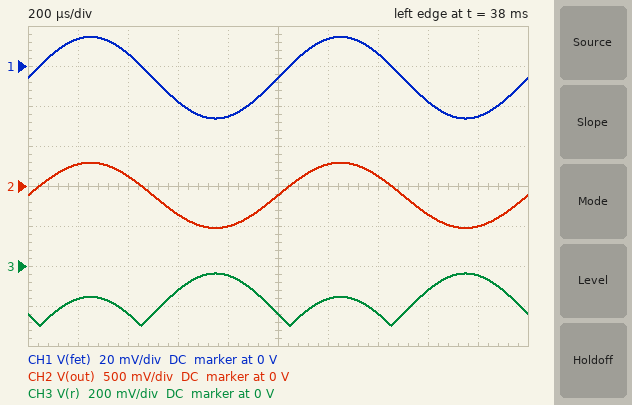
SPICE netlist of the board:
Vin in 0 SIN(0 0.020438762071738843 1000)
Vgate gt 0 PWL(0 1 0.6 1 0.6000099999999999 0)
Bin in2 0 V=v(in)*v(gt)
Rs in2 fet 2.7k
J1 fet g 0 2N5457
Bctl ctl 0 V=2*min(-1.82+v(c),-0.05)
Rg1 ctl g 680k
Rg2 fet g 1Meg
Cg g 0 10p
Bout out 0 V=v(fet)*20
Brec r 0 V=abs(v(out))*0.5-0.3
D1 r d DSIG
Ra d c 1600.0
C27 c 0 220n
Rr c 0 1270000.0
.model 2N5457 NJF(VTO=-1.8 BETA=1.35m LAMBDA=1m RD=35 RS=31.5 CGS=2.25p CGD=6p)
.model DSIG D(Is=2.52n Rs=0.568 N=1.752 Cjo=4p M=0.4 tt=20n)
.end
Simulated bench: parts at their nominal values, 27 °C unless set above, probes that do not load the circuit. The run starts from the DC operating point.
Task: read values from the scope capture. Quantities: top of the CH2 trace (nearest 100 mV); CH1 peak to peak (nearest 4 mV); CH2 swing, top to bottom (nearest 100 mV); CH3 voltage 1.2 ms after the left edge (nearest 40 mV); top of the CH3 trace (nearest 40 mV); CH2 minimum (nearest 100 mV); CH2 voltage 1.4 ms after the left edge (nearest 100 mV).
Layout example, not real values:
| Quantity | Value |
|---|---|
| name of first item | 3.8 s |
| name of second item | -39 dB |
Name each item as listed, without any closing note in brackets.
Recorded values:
| Quantity | Value |
|---|---|
| top of the CH2 trace | 300 mV |
| CH1 peak to peak | 40 mV |
| CH2 swing, top to bottom | 800 mV |
| CH3 voltage 1.2 ms after the left edge | -160 mV |
| top of the CH3 trace | -40 mV |
| CH2 minimum | -500 mV |
| CH2 voltage 1.4 ms after the left edge | 100 mV |
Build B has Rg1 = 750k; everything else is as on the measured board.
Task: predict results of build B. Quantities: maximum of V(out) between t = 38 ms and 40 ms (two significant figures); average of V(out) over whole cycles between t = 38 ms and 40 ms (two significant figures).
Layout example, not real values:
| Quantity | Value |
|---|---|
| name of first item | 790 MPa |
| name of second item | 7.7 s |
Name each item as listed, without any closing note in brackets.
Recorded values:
| Quantity | Value |
|---|---|
| maximum of V(out) between t = 38 ms and 40 ms | 300 mV |
| average of V(out) over whole cycles between t = 38 ms and 40 ms | -110 mV |
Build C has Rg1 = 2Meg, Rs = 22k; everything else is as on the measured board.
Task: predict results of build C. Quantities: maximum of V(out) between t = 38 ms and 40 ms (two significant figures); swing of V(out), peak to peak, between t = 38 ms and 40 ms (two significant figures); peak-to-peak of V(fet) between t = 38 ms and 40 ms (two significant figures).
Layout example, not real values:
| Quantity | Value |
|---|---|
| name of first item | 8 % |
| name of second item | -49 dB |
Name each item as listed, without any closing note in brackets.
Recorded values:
| Quantity | Value |
|---|---|
| maximum of V(out) between t = 38 ms and 40 ms | -3.9 mV |
| swing of V(out), peak to peak, between t = 38 ms and 40 ms | 25 mV |
| peak-to-peak of V(fet) between t = 38 ms and 40 ms | 1.3 mV |
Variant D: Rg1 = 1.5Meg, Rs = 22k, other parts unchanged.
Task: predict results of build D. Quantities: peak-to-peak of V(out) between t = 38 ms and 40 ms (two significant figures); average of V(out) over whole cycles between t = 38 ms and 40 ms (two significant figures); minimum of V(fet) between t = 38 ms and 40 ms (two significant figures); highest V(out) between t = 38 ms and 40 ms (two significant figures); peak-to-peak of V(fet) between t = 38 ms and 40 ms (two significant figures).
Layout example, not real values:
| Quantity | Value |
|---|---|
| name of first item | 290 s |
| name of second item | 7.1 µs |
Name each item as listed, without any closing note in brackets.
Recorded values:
| Quantity | Value |
|---|---|
| peak-to-peak of V(out) between t = 38 ms and 40 ms | 41 mV |
| average of V(out) over whole cycles between t = 38 ms and 40 ms | -32 mV |
| minimum of V(fet) between t = 38 ms and 40 ms | -2.6 mV |
| highest V(out) between t = 38 ms and 40 ms | -12 mV |
| peak-to-peak of V(fet) between t = 38 ms and 40 ms | 2.0 mV |
